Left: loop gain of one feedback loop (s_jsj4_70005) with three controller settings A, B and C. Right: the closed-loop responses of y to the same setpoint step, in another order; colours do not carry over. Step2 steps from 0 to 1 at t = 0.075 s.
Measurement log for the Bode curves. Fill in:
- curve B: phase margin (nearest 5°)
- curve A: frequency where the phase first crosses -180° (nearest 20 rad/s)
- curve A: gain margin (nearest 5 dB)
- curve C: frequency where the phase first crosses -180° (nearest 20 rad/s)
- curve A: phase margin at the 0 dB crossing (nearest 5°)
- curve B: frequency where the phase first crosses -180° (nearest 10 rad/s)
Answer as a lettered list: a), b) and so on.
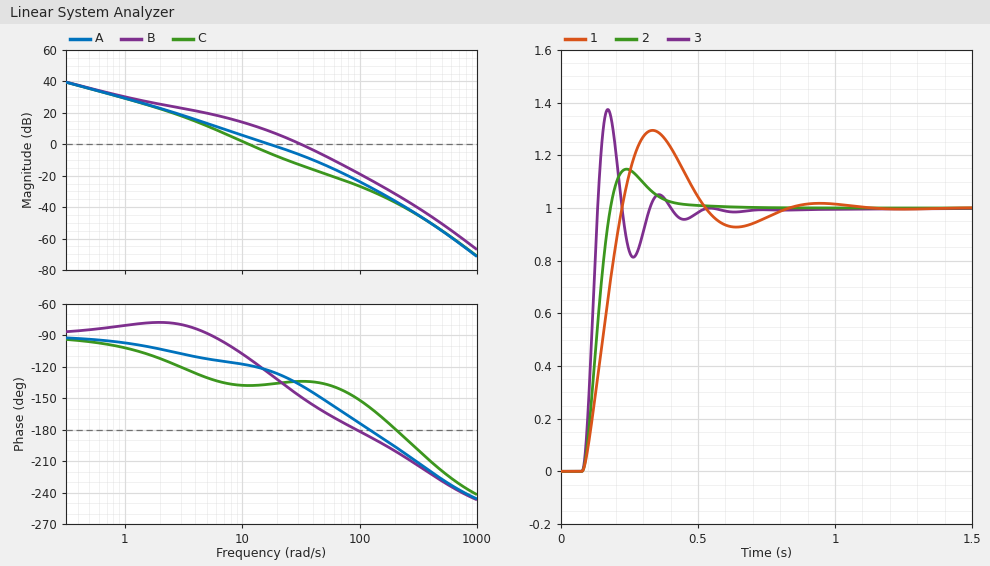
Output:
a) 30°
b) 120 rad/s
c) 25 dB
d) 200 rad/s
e) 55°
f) 90 rad/s
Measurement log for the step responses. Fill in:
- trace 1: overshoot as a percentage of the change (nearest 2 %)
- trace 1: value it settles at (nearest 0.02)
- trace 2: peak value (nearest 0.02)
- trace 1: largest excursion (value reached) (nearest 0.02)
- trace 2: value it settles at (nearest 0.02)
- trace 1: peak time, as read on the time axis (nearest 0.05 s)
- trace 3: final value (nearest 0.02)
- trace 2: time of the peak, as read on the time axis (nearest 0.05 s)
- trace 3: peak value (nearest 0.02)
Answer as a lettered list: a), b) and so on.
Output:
a) 30 %
b) 1.00
c) 1.14
d) 1.30
e) 1.00
f) 0.35 s
g) 1.00
h) 0.25 s
i) 1.38
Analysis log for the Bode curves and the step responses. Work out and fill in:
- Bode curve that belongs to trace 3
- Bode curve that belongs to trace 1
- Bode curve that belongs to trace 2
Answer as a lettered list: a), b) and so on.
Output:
a) B
b) C
c) A
